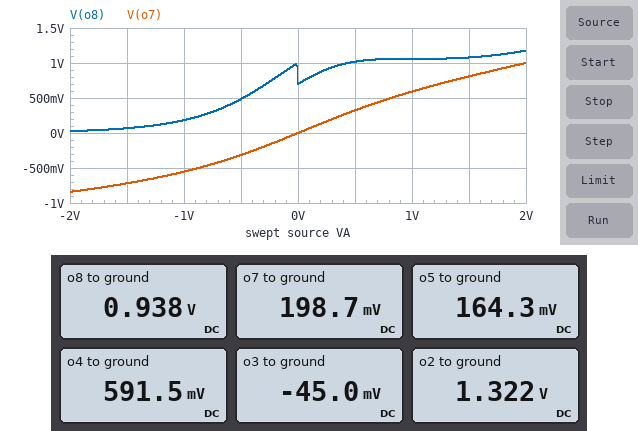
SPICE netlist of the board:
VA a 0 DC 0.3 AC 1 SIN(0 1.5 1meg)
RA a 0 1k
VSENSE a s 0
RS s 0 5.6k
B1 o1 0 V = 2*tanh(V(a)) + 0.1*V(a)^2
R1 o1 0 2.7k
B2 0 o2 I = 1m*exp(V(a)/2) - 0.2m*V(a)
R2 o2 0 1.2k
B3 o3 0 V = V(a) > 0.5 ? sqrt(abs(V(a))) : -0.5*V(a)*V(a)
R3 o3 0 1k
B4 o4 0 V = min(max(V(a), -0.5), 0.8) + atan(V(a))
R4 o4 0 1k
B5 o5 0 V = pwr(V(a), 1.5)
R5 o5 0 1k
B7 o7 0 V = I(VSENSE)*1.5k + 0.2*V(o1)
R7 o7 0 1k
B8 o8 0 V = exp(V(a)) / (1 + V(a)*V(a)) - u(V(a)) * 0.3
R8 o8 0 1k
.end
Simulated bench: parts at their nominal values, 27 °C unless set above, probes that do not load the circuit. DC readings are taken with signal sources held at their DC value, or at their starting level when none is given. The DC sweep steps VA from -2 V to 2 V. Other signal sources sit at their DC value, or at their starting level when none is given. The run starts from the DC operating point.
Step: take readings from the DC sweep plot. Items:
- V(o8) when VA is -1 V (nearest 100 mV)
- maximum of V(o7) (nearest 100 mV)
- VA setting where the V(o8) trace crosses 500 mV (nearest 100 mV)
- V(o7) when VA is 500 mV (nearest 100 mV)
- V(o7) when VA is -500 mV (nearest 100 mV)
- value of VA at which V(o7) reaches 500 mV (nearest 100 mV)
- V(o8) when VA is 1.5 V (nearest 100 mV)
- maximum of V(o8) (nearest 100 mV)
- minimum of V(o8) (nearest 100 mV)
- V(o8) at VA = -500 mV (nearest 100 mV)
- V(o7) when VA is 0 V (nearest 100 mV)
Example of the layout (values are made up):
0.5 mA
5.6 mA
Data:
200 mV
1.0 V
-500 mV
300 mV
-300 mV
800 mV
1.1 V
1.2 V
0 V
500 mV
0 V
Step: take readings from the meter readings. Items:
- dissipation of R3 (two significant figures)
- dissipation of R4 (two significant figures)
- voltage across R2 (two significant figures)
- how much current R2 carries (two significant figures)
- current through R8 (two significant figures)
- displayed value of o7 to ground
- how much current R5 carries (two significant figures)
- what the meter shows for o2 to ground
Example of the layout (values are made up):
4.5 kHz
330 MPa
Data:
2.0 µW
350 µW
1.3 V
1.1 mA
940 µA
198.7 mV
160 µA
1.322 V
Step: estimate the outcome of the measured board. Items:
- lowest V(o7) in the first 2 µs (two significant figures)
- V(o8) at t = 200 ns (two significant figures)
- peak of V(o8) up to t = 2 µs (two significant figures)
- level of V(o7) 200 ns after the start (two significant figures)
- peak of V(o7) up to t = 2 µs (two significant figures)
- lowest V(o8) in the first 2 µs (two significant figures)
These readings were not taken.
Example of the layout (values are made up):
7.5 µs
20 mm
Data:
-720 mV
1.1 V
1.1 V
780 mV
810 mV
69 mV
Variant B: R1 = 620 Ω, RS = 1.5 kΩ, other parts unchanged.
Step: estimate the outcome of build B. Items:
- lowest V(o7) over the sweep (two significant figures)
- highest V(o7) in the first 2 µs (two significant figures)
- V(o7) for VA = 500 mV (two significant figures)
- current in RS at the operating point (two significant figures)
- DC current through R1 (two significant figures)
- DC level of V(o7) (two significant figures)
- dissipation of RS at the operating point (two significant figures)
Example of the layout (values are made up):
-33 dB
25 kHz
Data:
-2.3 V
1.9 V
690 mV
200 µA
950 µA
420 mV
60 µW
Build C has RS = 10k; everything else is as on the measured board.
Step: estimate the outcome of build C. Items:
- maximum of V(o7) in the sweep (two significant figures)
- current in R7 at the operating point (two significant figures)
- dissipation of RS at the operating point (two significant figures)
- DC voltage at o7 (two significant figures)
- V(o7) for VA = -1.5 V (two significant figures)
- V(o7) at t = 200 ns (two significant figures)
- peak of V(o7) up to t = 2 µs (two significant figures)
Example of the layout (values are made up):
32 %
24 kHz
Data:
770 mV
160 µA
9.0 µW
160 mV
-540 mV
610 mV
630 mV
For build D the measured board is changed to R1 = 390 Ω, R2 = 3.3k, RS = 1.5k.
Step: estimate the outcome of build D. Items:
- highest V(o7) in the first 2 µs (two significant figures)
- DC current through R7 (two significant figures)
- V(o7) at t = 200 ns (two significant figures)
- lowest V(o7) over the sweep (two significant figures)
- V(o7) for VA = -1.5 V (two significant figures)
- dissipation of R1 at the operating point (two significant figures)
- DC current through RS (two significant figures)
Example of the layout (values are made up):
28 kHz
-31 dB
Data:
1.9 V
420 µA
1.8 V
-2.3 V
-1.8 V
900 µW
200 µA
